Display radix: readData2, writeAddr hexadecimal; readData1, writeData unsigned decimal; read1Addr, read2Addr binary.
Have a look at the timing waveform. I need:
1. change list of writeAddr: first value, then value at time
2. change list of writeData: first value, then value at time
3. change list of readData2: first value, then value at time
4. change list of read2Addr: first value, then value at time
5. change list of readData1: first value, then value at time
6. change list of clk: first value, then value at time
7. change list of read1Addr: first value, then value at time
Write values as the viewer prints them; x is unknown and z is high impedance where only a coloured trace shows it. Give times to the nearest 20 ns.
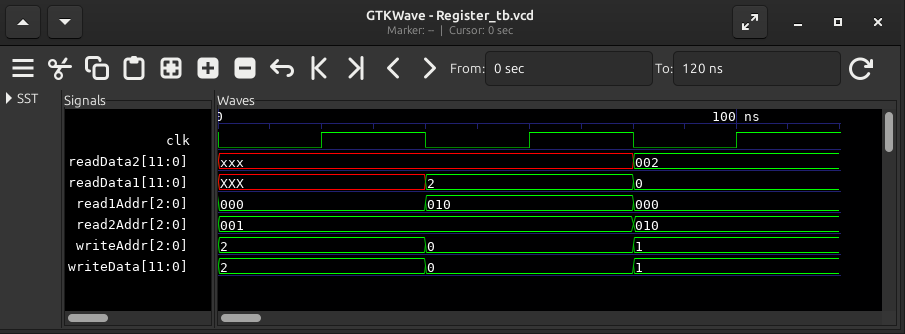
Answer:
2, 0 at 40 ns, 1 at 80 ns
2, 0 at 40 ns, 1 at 80 ns
xxx, 002 at 80 ns
001, 010 at 80 ns
XXX, 2 at 40 ns, 0 at 80 ns
0, 1 at 20 ns, 0 at 40 ns, 1 at 60 ns, 0 at 80 ns, 1 at 100 ns
000, 010 at 40 ns, 000 at 80 ns
